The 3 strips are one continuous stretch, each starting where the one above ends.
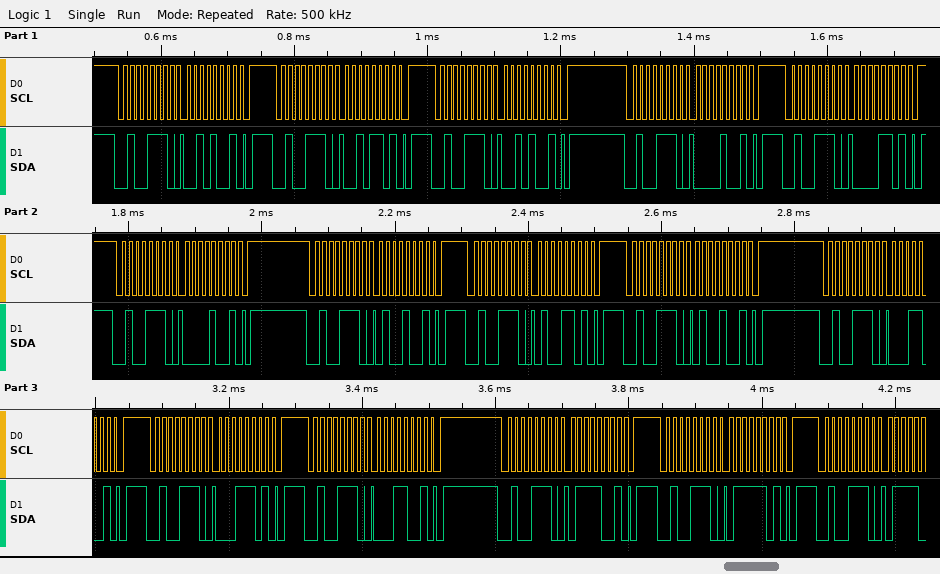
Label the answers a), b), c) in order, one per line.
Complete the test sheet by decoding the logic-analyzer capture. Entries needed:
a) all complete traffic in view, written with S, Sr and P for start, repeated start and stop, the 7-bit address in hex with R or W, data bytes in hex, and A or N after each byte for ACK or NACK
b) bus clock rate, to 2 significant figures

a) S 27W A 29 A P S 27W A 2D A P S 27W A 29 A P S 27W A 09 A P S 27W A 0D A P S 27W A 09 A P S 27W A 49 A P S 27W A 4D A P S 27W A 49 A P S 27W A 19 A P S 27W A 1D A P S 27W A 19 A P S 27W A 79 A P S 27W A 7D A P S 27W A
b) 100 kHz
